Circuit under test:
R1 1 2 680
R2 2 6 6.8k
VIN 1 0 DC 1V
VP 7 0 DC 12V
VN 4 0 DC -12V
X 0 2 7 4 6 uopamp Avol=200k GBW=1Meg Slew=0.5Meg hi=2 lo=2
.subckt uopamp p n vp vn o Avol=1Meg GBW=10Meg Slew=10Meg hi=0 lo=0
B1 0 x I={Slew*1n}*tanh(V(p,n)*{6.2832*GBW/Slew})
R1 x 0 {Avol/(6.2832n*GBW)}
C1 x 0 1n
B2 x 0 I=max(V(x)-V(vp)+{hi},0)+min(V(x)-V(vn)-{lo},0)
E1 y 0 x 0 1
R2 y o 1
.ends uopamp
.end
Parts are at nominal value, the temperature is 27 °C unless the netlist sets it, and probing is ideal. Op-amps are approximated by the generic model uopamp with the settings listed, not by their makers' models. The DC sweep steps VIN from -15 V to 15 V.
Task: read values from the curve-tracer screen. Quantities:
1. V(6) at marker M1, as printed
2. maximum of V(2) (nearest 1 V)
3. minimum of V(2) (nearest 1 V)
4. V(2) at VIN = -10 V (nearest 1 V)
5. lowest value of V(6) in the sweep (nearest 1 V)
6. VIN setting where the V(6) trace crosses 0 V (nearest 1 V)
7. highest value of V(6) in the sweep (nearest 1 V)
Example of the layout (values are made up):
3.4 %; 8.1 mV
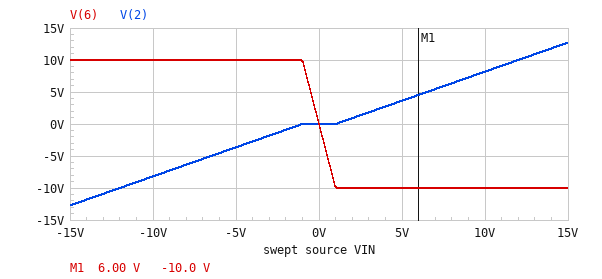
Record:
-10.0 V; 13 V; -13 V; -8 V; -10 V; 0 V; 10 V
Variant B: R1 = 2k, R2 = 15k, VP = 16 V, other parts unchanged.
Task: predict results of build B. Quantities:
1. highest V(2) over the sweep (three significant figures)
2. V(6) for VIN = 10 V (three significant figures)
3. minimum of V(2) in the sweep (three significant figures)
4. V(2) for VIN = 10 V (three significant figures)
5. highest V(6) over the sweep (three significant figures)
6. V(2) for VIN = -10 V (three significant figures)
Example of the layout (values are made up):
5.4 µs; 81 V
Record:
12.1 V; -10.0 V; -11.6 V; 7.65 V; 14.0 V; -7.18 V
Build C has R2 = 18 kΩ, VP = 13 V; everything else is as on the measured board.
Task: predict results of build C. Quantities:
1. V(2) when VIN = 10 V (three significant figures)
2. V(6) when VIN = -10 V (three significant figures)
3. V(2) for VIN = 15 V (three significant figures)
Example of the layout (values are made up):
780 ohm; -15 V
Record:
9.27 V; 11.0 V; 14.1 V
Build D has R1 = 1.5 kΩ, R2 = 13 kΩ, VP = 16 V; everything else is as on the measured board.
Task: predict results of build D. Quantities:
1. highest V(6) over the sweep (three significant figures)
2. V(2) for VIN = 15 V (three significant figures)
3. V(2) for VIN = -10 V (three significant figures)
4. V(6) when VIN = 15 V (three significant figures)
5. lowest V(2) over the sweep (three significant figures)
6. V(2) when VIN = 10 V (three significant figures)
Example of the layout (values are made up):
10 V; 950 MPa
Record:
14.0 V; 12.4 V; -7.52 V; -10.0 V; -12.0 V; 7.93 V
